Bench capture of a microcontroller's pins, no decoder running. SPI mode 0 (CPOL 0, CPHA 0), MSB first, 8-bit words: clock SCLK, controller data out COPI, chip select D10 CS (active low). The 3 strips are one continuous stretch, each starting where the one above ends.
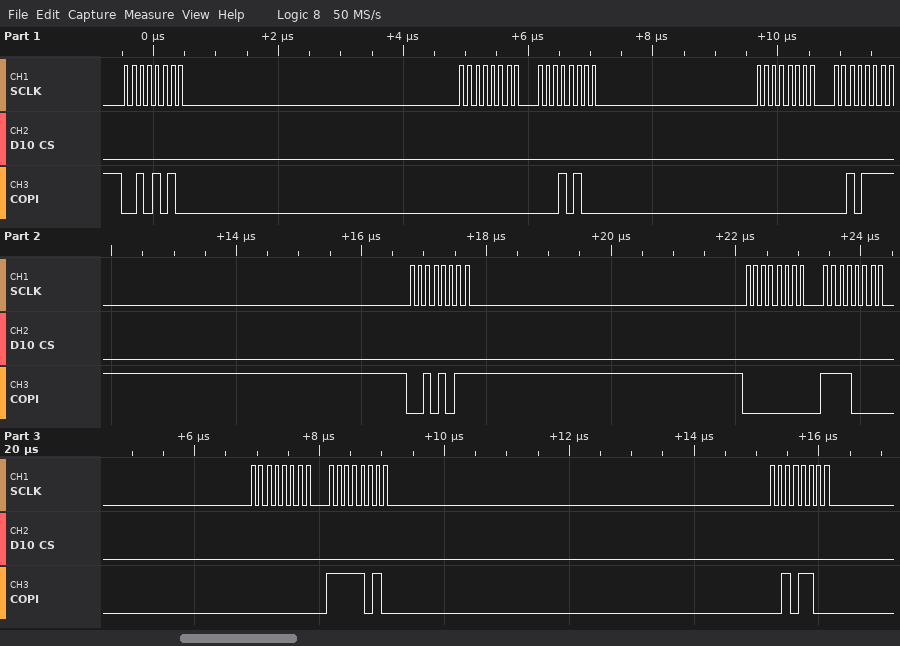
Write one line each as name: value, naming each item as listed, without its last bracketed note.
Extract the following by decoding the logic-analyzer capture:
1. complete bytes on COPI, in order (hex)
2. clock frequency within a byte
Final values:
complete bytes on COPI, in order: 2A 00 14 00 2F 2B 00 F0 00 FA 2C
clock frequency within a byte: 8 MHz
